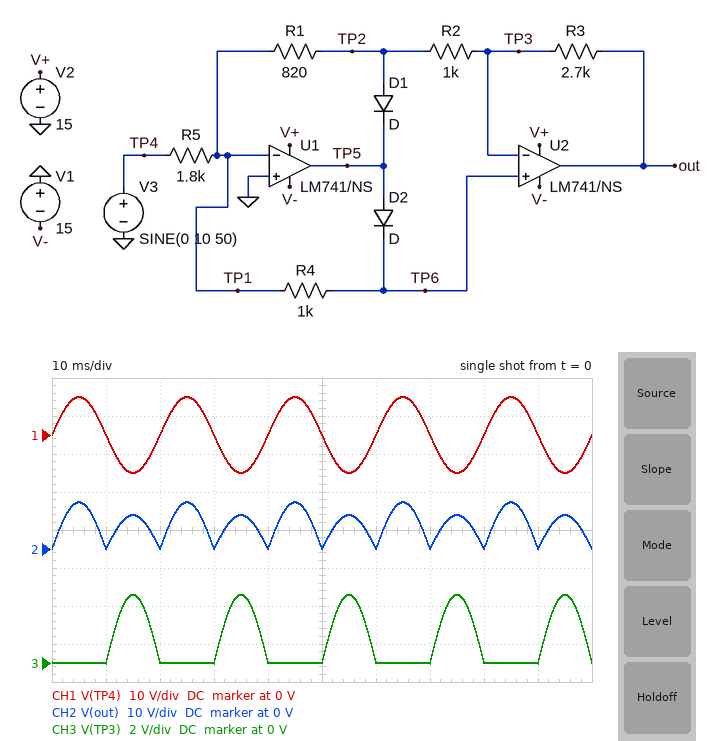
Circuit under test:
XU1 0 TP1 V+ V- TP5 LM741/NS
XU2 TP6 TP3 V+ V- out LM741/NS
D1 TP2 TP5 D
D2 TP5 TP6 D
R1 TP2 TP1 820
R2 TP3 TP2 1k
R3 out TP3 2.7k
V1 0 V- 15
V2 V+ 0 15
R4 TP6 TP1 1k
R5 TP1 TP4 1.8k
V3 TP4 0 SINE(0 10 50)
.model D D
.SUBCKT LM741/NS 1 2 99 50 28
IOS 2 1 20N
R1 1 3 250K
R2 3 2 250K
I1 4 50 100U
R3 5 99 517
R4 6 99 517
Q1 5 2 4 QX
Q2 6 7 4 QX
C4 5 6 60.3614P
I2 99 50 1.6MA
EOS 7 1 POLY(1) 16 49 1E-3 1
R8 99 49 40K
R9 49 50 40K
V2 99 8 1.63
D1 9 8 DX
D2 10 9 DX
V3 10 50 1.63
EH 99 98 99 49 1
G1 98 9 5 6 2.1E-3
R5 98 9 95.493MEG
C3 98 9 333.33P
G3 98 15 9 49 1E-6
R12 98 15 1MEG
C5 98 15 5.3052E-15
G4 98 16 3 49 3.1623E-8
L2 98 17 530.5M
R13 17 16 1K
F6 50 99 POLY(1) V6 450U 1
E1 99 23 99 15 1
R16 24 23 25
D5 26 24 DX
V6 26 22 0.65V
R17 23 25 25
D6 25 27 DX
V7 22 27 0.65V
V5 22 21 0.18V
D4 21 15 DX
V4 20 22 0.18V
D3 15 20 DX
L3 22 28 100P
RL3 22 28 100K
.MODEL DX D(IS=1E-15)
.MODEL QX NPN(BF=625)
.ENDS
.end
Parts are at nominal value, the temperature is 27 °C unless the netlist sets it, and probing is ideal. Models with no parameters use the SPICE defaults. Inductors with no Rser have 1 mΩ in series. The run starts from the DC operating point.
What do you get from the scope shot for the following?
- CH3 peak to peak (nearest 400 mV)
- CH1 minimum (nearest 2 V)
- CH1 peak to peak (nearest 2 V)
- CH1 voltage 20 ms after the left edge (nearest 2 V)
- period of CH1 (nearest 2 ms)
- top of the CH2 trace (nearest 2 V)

3.6 V
-10 V
20 V
0 V
20 ms
12 V
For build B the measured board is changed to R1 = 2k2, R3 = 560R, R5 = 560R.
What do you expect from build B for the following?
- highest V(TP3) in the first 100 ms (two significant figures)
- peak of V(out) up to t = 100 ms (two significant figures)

12 V
14 V
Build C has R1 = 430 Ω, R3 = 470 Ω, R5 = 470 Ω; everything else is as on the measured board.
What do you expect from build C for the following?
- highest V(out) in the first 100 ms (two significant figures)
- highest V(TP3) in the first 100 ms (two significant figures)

14 V
10 V
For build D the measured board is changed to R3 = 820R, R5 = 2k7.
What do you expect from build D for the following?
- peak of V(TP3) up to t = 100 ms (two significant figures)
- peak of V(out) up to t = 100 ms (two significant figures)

2.4 V
3.5 V
